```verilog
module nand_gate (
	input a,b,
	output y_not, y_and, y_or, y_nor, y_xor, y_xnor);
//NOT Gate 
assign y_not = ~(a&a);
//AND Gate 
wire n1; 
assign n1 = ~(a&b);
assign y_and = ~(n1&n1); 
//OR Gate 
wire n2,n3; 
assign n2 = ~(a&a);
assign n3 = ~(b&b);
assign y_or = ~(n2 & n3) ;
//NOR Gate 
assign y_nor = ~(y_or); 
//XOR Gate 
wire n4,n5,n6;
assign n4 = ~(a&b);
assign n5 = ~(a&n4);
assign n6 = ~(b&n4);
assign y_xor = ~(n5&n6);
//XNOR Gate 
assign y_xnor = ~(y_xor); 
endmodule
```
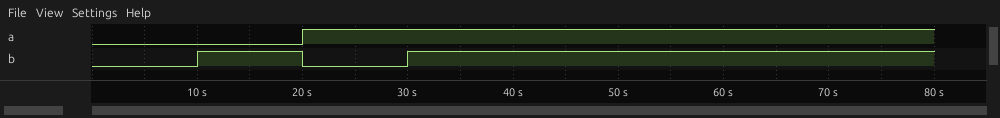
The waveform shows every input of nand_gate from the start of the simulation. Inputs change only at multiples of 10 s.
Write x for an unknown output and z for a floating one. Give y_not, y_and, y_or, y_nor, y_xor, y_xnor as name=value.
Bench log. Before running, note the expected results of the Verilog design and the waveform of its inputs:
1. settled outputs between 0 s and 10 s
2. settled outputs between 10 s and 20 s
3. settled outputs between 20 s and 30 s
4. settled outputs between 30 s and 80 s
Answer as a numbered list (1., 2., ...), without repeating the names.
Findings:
1. y_not=1, y_and=0, y_or=0, y_nor=1, y_xor=0, y_xnor=1
2. y_not=1, y_and=0, y_or=1, y_nor=0, y_xor=1, y_xnor=0
3. y_not=0, y_and=0, y_or=1, y_nor=0, y_xor=1, y_xnor=0
4. y_not=0, y_and=1, y_or=1, y_nor=0, y_xor=0, y_xnor=1
